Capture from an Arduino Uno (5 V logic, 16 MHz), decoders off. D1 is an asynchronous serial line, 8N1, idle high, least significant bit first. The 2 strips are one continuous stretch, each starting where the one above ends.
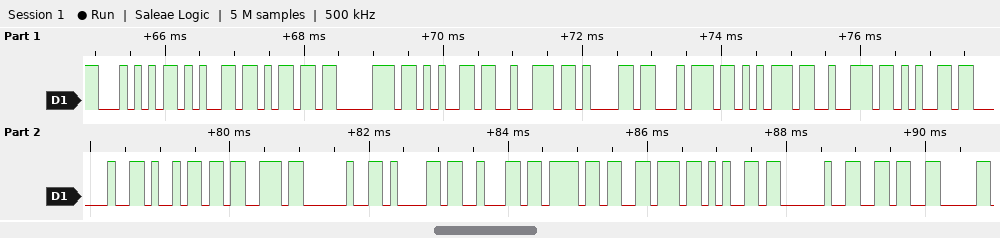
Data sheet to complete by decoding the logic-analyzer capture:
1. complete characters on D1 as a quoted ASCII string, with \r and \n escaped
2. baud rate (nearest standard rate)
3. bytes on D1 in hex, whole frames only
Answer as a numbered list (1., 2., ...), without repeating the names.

1. "Temperature is above 6"
2. 9600 baud
3. 54 65 6D 70 65 72 61 74 75 72 65 20 69 73 20 61 62 6F 76 65 20 36
